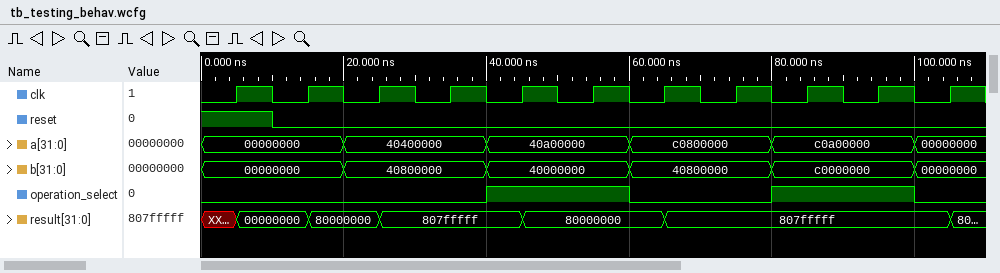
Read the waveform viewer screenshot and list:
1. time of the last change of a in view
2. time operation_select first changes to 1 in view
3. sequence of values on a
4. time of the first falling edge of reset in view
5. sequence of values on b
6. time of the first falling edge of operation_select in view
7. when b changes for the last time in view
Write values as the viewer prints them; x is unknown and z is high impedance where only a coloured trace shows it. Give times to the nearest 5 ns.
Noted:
100 ns
40 ns
00000000, 40400000, 40a00000, c0800000, c0a00000, 00000000
10 ns
00000000, 40800000, 40000000, 40800000, c0000000, 00000000
60 ns
100 ns
